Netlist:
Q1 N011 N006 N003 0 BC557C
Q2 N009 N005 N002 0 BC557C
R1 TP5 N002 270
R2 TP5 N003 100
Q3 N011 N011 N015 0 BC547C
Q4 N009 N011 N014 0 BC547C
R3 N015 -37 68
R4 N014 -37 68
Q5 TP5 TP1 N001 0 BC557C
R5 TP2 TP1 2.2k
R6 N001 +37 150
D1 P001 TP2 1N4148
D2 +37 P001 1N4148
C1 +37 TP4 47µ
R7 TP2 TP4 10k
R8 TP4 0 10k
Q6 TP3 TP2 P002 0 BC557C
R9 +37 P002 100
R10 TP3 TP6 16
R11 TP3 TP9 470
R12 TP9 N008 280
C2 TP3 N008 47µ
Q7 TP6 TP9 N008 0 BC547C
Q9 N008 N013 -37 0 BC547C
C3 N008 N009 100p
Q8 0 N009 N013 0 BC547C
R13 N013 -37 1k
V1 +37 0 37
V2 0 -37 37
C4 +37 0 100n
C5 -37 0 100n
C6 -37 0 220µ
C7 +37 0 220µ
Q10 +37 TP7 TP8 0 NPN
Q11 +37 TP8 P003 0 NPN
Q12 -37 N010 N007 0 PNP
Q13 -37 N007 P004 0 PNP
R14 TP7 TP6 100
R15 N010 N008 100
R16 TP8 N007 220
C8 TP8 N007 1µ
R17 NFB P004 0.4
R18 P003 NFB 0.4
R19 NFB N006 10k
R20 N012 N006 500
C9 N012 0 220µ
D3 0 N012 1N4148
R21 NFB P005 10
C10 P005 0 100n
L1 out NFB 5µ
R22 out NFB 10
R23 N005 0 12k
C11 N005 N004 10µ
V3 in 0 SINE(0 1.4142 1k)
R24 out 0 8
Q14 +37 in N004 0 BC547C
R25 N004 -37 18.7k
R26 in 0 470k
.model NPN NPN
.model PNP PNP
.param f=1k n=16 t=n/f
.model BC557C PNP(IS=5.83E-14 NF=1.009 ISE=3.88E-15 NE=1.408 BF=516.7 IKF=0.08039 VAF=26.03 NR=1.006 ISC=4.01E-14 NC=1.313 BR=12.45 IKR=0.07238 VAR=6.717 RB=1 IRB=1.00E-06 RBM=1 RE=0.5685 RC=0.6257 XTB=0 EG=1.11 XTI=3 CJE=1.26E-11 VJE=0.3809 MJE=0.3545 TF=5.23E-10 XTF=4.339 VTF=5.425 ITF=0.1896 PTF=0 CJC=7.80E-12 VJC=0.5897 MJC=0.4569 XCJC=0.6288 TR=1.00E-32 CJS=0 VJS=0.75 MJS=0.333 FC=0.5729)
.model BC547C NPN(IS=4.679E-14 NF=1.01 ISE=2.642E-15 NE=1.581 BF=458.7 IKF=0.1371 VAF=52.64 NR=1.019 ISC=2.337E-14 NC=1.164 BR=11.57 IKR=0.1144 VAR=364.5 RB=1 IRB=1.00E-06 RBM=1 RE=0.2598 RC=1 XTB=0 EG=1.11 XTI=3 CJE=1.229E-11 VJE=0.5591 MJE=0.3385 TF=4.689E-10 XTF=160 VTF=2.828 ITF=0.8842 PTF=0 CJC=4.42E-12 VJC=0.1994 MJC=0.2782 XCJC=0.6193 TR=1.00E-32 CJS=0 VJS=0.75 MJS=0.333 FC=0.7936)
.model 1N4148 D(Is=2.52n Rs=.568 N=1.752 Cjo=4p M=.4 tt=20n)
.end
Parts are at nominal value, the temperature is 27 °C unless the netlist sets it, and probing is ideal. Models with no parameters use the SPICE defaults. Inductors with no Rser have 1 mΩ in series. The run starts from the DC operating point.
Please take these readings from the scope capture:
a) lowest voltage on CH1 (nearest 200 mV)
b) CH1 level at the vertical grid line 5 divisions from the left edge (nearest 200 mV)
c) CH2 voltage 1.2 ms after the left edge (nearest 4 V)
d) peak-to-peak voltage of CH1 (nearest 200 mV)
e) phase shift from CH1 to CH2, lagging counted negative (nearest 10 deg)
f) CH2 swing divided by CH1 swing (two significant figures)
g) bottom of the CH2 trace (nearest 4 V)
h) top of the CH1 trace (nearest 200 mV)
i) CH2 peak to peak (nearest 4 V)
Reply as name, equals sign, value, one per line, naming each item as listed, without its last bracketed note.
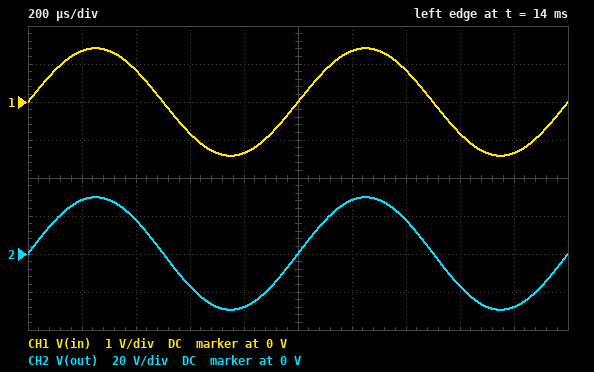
lowest voltage on CH1 = -1.4 V
CH1 level at the vertical grid line 5 divisions from the left edge = 0 V
CH2 voltage 1.2 ms after the left edge = 28 V
peak-to-peak voltage of CH1 = 2.8 V
phase shift from CH1 to CH2, lagging counted negative = 0 deg
CH2 swing divided by CH1 swing = 21
bottom of the CH2 trace = -28 V
top of the CH1 trace = 1.4 V
CH2 peak to peak = 60 V
